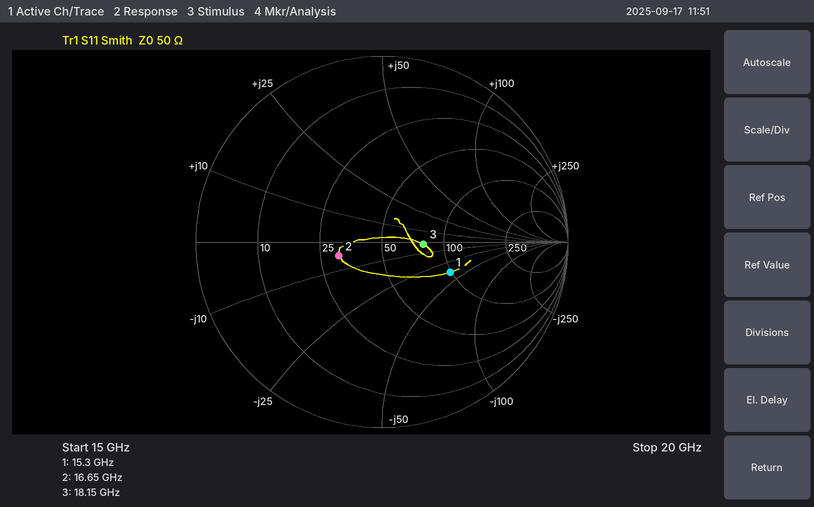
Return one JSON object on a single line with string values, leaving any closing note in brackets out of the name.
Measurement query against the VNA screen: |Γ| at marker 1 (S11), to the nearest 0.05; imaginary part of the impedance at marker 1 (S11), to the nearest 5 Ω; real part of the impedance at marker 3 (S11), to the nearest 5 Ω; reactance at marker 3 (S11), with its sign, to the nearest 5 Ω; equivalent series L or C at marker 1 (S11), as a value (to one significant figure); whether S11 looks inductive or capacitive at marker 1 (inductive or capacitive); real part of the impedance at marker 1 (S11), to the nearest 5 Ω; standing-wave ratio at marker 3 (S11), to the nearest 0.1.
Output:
{"|Γ| at marker 1 (S11), to the nearest 0.05": "0.40", "imaginary part of the impedance at marker 1 (S11), to the nearest 5 Ω": "-40 Ω", "real part of the impedance at marker 3 (S11), to the nearest 5 Ω": "80 Ω", "reactance at marker 3 (S11), with its sign, to the nearest 5 Ω": "0 Ω", "equivalent series L or C at marker 1 (S11), as a value": "300 fF", "whether S11 looks inductive or capacitive at marker 1": "capacitive", "real part of the impedance at marker 1 (S11), to the nearest 5 Ω": "100 Ω", "standing-wave ratio at marker 3 (S11), to the nearest 0.1": "1.6"}
